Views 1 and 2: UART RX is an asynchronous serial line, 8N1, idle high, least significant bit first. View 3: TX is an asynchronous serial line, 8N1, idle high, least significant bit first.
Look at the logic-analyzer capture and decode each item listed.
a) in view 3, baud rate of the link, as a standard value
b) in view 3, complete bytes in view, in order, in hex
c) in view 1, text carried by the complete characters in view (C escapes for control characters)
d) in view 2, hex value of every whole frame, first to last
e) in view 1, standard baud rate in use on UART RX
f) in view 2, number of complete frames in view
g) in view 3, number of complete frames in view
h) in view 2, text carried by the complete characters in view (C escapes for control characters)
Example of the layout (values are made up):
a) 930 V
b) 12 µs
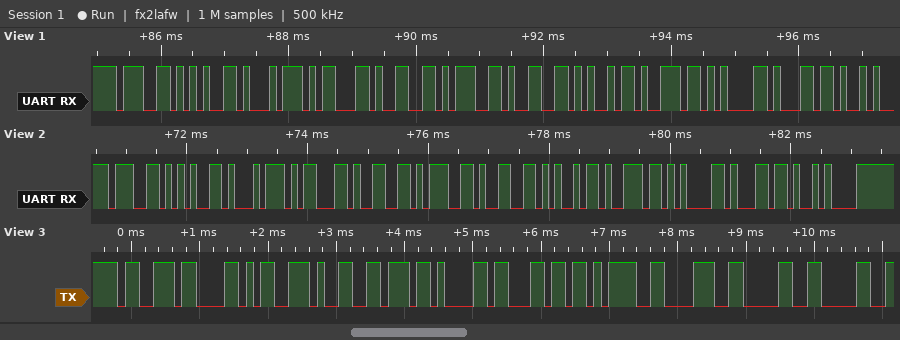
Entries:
a) 9600 baud
b) 0x73 0x58 0x2E 0x76 0x61 0x6C 0x3D 0x38 0x30 0x30
c) "getcfgfinal"
d) 0x67 0x65 0x74 0x63 0x66 0x67 0x66 0x69 0x6E 0x61 0x6C 0x0A
e) 9600 baud
f) 12
g) 10
h) "getcfgfinal\n"
